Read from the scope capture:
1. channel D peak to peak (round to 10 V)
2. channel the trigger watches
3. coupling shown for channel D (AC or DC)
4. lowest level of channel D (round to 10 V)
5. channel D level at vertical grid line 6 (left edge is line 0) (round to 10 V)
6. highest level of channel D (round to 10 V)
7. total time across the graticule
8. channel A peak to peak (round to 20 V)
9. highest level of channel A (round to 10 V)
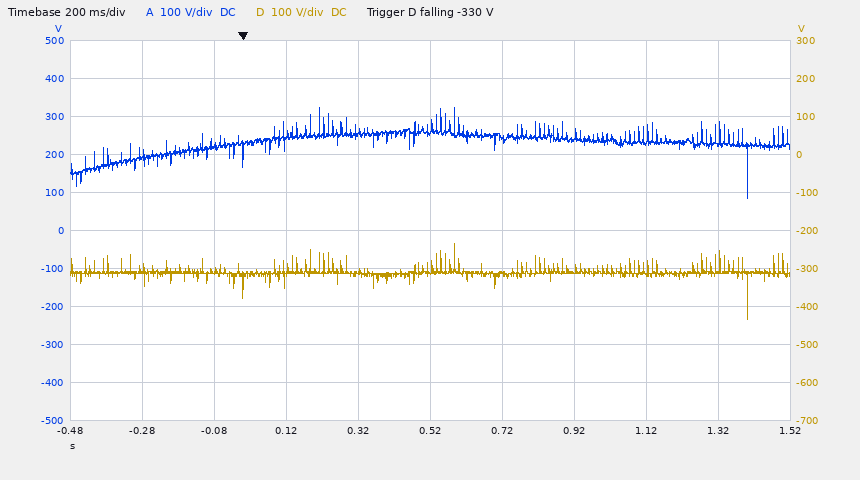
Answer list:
200 V
channel D
DC
-430 V
-310 V
-230 V
2 s
240 V
320 V
